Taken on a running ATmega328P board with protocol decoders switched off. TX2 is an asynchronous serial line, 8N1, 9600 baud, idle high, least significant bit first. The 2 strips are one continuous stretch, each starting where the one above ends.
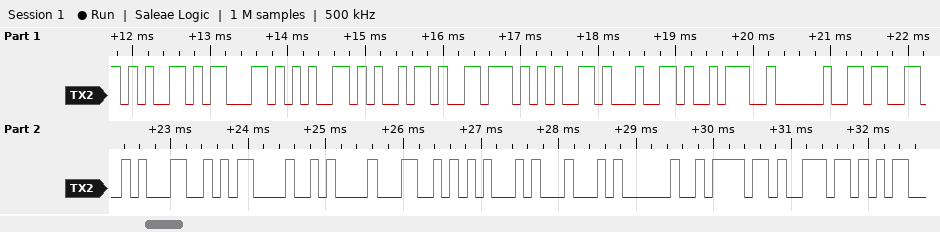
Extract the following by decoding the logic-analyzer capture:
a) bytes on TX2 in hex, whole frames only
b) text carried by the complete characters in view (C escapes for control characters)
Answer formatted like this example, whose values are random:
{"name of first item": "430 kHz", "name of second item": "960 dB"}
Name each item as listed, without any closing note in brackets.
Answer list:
{"bytes on TX2 in hex, whole frames only": "65 63 65 69 76 65 64 3A 20 33 31 0D 0A 4C 45 44 20 6F 6E", "text carried by the complete characters in view": "\"eceived: 31\\r\\nLED on\""}
